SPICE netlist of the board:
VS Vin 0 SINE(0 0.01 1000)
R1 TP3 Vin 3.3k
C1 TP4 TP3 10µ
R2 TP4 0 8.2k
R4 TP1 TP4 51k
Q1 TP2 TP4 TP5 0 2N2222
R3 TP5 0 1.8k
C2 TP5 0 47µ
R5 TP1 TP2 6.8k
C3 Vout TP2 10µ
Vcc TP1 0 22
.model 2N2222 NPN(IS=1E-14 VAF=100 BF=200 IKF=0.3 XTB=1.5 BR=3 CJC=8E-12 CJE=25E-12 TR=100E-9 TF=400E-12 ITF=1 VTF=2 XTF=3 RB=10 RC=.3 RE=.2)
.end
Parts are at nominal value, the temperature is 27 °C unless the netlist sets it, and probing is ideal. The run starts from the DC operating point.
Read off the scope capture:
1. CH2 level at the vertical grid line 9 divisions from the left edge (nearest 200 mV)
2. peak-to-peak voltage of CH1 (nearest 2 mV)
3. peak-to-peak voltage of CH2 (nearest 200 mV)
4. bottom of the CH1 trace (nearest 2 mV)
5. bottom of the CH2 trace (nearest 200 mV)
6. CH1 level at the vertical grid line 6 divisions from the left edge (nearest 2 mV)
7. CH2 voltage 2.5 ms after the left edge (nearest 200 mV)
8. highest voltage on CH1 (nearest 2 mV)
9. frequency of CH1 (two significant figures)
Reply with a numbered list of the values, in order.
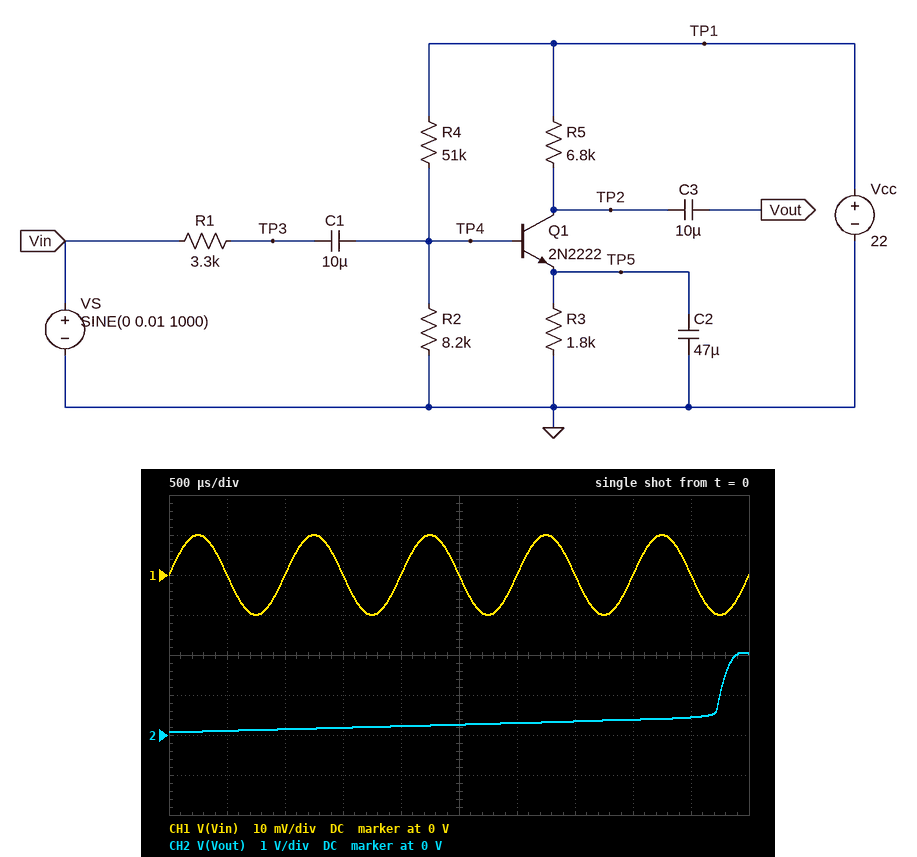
1. 400 mV
2. 20 mV
3. 2.0 V
4. -10 mV
5. 0 V
6. 0 V
7. 200 mV
8. 10 mV
9. 1.0 kHz
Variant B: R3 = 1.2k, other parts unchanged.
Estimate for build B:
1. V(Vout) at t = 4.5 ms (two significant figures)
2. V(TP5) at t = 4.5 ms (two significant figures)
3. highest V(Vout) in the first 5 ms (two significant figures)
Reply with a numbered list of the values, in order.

1. 430 mV
2. 300 mV
3. 970 mV
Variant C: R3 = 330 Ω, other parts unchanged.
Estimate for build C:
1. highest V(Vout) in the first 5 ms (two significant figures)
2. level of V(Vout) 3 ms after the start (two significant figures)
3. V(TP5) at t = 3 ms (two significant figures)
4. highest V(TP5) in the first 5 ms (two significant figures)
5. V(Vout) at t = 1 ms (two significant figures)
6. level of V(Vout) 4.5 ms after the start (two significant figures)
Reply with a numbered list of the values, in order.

1. 410 mV
2. 280 mV
3. 190 mV
4. 300 mV
5. 140 mV
6. 380 mV
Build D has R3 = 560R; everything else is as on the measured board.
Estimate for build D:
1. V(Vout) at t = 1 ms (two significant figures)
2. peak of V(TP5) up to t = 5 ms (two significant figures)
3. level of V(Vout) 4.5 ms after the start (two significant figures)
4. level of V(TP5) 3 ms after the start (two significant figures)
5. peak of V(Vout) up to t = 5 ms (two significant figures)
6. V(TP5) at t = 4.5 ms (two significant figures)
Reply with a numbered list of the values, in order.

1. 140 mV
2. 320 mV
3. 400 mV
4. 200 mV
5. 450 mV
6. 290 mV
